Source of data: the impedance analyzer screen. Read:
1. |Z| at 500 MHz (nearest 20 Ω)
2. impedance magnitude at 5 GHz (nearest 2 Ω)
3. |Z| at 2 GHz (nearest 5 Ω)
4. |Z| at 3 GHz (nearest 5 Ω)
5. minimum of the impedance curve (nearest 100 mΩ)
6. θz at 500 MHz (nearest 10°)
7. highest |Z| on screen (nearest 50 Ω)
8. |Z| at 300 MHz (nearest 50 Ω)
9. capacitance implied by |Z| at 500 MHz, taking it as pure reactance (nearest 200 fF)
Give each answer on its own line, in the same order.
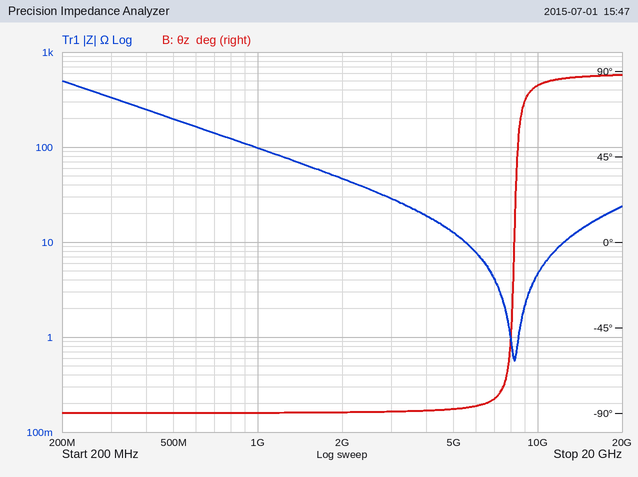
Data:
200 Ω
12 Ω
45 Ω
30 Ω
600 mΩ
-90°
500 Ω
350 Ω
1.6 pF
